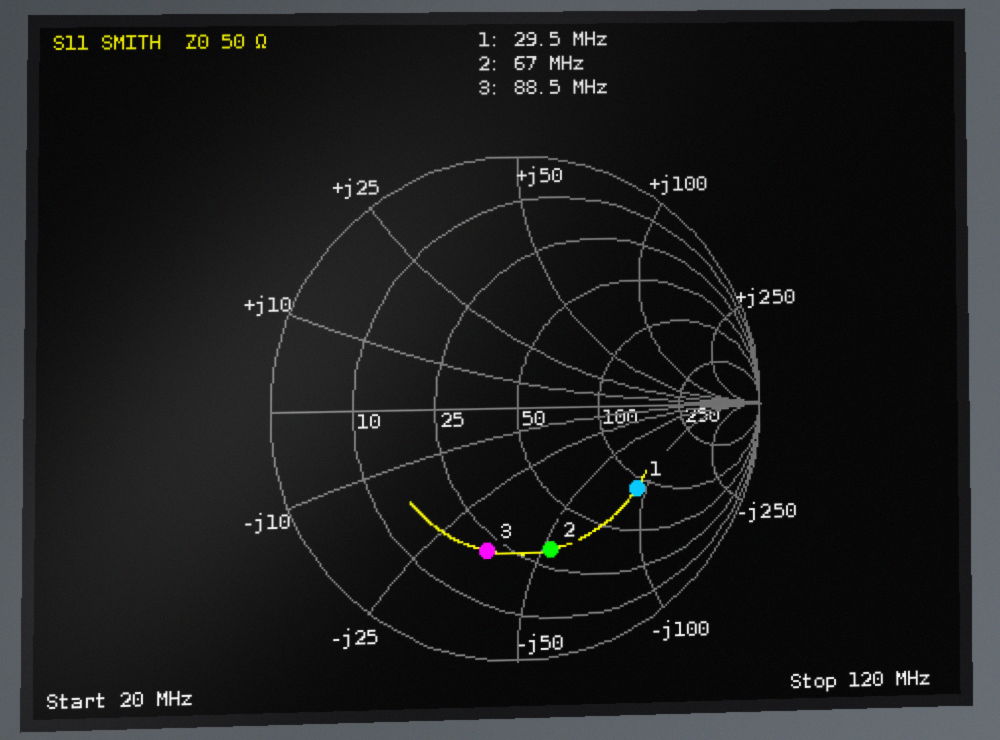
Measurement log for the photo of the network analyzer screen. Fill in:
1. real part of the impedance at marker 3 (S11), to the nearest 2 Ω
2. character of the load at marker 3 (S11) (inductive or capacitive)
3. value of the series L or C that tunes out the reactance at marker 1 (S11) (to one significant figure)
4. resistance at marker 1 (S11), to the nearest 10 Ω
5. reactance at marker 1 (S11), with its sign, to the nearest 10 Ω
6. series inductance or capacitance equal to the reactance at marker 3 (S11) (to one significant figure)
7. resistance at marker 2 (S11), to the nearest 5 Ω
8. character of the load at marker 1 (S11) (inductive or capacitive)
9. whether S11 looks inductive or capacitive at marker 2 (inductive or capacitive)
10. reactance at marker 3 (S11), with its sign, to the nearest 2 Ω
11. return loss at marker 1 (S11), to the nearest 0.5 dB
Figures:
22 Ω
capacitive
500 nH
90 Ω
-90 Ω
50 pF
30 Ω
capacitive
capacitive
-36 Ω
4.5 dB
